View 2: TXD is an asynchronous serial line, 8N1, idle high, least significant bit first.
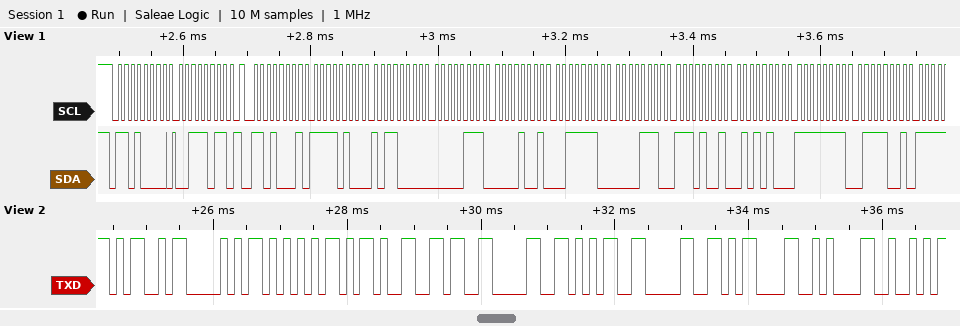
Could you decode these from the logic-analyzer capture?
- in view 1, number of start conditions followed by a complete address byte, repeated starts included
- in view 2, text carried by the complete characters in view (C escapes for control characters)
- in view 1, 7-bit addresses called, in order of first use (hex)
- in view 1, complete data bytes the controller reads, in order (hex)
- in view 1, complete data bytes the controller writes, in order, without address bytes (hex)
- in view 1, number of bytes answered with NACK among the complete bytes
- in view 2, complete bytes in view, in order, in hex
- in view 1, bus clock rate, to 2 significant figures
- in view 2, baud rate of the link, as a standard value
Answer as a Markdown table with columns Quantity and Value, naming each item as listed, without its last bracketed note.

| Quantity | Value |
|---|---|
| in view 1, number of start conditions followed by a complete address byte, repeated starts included | 2 |
| in view 2, text carried by the complete characters in view | "MPU-6050\r\nR" |
| in view 1, 7-bit addresses called, in order of first use | 0x68 |
| in view 1, complete data bytes the controller reads, in order | F4 B0 07 09 3E 0E E9 54 FF 79 |
| in view 1, complete data bytes the controller writes, in order, without address bytes | 3B |
| in view 1, number of bytes answered with NACK among the complete bytes | 0 |
| in view 2, complete bytes in view, in order, in hex | 4D 50 55 2D 36 30 35 30 0D 0A 52 |
| in view 1, bus clock rate, to 2 significant figures | 100 kHz |
| in view 2, baud rate of the link, as a standard value | 9600 baud |
